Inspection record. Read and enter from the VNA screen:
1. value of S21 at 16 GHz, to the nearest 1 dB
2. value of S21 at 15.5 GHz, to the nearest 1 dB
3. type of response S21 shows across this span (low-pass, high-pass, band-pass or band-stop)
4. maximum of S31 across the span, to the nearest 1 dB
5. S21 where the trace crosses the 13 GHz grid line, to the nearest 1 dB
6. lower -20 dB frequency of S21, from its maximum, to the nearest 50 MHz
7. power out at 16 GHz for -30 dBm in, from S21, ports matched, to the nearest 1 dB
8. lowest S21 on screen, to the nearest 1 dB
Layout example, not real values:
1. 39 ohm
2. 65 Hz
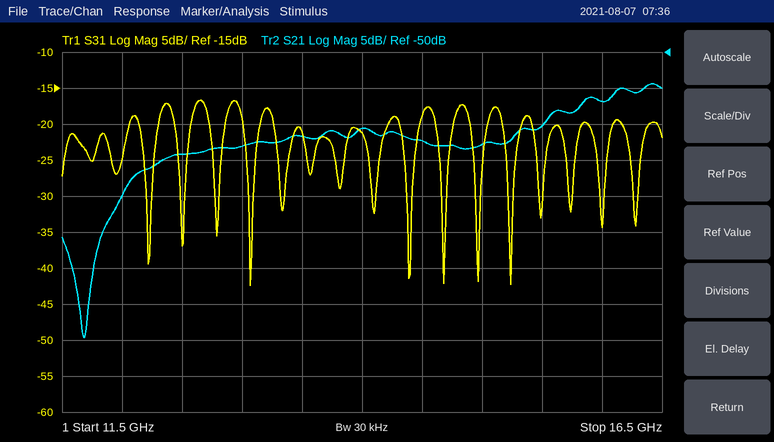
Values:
1. -57 dB
2. -60 dB
3. high-pass
4. -17 dB
5. -63 dB
6. 11.85 GHz
7. -87 dBm
8. -90 dB
